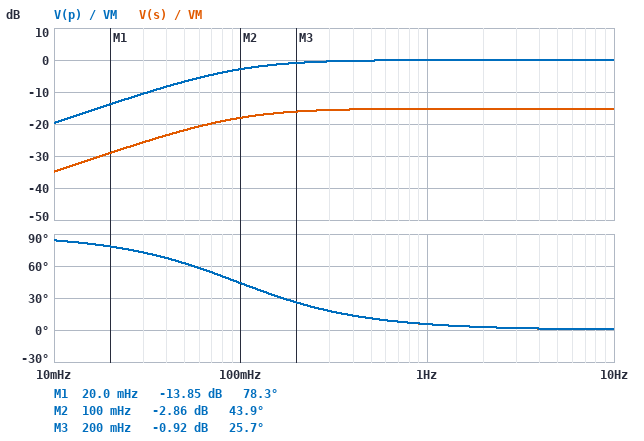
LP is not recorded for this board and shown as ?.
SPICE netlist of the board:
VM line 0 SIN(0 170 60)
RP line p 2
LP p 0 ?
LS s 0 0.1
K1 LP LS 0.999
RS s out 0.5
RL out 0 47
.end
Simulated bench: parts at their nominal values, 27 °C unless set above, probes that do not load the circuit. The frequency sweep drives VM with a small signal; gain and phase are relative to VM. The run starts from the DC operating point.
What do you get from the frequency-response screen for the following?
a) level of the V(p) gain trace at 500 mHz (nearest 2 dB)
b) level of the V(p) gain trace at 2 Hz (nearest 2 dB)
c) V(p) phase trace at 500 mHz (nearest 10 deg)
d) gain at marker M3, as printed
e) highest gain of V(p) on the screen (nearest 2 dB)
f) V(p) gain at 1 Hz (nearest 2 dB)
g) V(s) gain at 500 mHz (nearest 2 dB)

0 dB
0 dB
10 deg
-0.92 dB
0 dB
0 dB
-16 dB
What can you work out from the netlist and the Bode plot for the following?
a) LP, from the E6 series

3.3 H
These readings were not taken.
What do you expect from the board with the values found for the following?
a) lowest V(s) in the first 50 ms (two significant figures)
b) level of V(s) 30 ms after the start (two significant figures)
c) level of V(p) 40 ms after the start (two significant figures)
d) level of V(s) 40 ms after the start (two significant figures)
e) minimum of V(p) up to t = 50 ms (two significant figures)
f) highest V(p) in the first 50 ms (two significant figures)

-30 V
-28 V
99 V
17 V
-170 V
170 V
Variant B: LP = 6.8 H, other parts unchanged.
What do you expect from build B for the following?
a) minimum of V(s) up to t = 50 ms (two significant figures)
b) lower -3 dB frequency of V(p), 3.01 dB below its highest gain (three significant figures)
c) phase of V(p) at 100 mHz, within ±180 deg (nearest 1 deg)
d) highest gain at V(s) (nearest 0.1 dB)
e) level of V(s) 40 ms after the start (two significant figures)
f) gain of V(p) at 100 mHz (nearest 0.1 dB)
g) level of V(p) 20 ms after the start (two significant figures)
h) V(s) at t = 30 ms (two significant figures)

-21 V
46.8 mHz
25 deg
-18.3 dB
12 V
-0.9 dB
160 V
-20 V
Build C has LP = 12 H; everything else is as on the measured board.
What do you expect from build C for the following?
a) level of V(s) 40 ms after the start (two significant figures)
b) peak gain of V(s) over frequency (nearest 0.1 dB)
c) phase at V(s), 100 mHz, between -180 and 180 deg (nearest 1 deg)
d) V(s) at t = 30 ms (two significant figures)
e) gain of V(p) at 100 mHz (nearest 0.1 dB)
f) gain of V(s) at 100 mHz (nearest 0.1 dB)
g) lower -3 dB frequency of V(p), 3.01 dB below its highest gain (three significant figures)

9.1 V
-20.8 dB
15 deg
-15 V
-0.3 dB
-21.1 dB
26.5 mHz
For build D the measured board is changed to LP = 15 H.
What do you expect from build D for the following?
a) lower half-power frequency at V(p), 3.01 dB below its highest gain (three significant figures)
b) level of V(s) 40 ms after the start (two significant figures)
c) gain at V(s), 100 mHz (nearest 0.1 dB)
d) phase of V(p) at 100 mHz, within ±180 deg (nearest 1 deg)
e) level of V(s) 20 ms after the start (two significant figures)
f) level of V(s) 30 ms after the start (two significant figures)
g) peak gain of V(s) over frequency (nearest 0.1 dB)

21.2 mHz
8.2 V
-22.0 dB
12 deg
13 V
-13 V
-21.8 dB
